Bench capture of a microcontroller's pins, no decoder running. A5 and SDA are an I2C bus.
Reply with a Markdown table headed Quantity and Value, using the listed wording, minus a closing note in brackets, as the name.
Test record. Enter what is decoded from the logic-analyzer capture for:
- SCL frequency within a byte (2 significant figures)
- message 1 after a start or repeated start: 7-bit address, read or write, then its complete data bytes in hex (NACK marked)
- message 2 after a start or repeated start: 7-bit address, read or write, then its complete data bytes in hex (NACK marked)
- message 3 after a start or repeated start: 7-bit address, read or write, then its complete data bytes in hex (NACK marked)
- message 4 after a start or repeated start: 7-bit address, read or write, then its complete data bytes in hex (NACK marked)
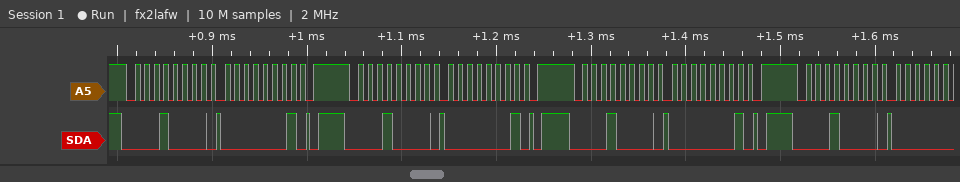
| Quantity | Value |
|---|---|
| SCL frequency within a byte | 100 kHz |
| message 1 after a start or repeated start: 7-bit address, read or write, then its complete data bytes in hex | 0x08 write: 01 |
| message 2 after a start or repeated start: 7-bit address, read or write, then its complete data bytes in hex | 0x08 write: 01 |
| message 3 after a start or repeated start: 7-bit address, read or write, then its complete data bytes in hex | 0x08 write: 01 |
| message 4 after a start or repeated start: 7-bit address, read or write, then its complete data bytes in hex | 0x08 write |
